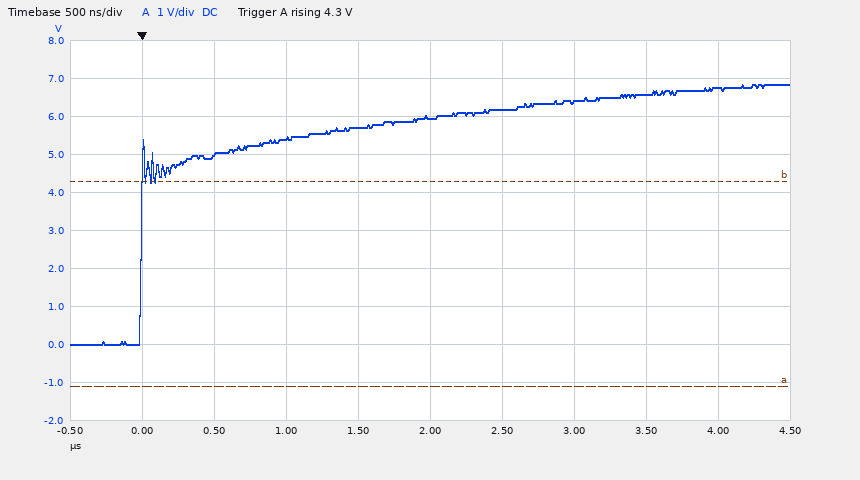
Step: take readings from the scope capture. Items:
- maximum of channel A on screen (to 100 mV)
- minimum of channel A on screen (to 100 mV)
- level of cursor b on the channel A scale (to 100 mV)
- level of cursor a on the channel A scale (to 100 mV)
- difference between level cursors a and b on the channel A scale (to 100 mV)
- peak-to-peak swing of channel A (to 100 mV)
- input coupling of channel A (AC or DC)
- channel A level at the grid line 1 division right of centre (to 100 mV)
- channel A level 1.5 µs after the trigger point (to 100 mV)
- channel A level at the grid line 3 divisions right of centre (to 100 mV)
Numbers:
6.8 V
0.0 V
4.3 V
-1.1 V
5.4 V
6.8 V
DC
6.2 V
5.7 V
6.6 V
